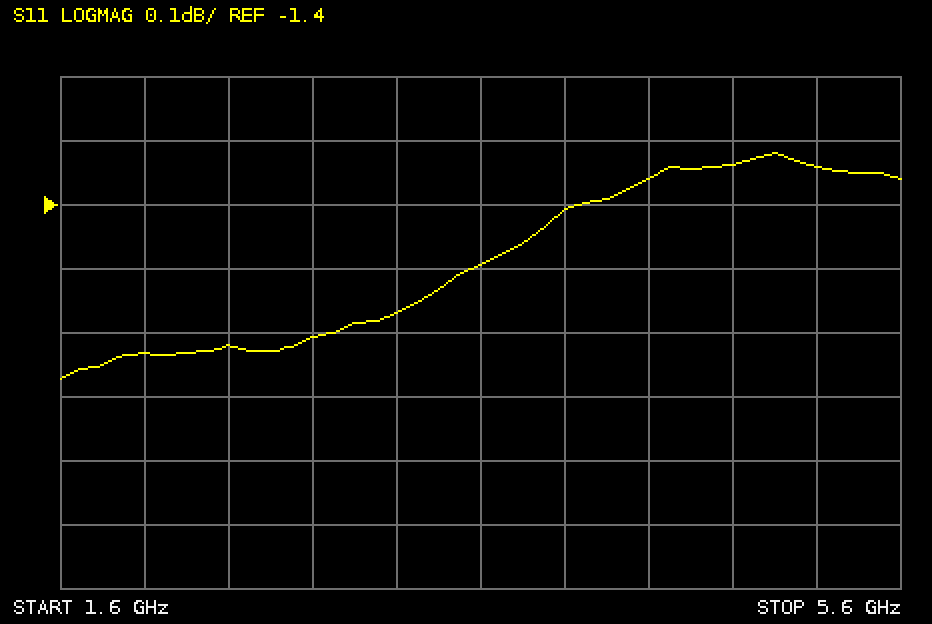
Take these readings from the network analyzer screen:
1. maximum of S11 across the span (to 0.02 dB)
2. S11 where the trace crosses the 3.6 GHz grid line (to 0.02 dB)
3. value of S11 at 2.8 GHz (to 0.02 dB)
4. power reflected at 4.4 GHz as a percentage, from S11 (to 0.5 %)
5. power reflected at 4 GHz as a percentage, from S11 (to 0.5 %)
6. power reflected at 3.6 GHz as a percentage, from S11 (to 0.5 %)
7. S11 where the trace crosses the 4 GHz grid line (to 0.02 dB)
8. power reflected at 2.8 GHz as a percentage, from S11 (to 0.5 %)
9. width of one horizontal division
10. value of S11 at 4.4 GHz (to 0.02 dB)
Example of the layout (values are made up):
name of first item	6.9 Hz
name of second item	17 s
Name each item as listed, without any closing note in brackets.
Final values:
maximum of S11 across the span	-1.32 dB
S11 where the trace crosses the 3.6 GHz grid line	-1.50 dB
value of S11 at 2.8 GHz	-1.60 dB
power reflected at 4.4 GHz as a percentage, from S11	73.0 %
power reflected at 4 GHz as a percentage, from S11	72.5 %
power reflected at 3.6 GHz as a percentage, from S11	71.0 %
S11 where the trace crosses the 4 GHz grid line	-1.40 dB
power reflected at 2.8 GHz as a percentage, from S11	69.0 %
width of one horizontal division	400 MHz
value of S11 at 4.4 GHz	-1.36 dB
